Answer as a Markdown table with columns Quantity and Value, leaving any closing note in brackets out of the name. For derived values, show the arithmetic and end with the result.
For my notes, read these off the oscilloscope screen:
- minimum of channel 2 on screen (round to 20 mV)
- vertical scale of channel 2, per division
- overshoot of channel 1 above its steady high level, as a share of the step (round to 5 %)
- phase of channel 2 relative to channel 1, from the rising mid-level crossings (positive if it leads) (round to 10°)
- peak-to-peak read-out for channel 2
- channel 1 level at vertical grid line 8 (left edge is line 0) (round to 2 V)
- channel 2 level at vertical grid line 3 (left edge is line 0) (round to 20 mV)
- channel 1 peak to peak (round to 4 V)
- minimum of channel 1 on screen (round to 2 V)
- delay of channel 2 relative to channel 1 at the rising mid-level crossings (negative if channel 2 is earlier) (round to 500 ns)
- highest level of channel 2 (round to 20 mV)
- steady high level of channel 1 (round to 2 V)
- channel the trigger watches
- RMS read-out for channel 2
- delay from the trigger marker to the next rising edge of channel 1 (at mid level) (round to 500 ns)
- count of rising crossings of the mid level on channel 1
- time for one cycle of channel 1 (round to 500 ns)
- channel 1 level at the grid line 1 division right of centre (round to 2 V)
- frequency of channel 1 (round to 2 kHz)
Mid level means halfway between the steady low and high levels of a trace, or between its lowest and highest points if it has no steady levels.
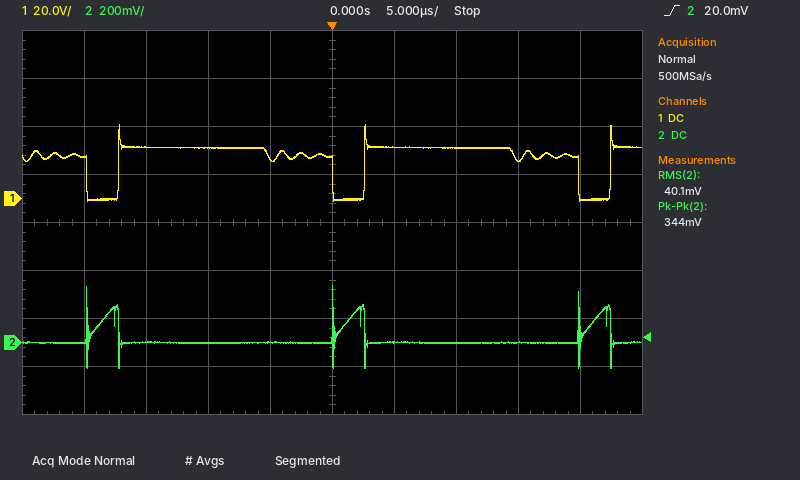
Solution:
| Quantity | Value |
|---|---|
| minimum of channel 2 on screen | -100 mV |
| vertical scale of channel 2, per division | 200 mV |
| overshoot of channel 1 above its steady high level, as a share of the step | 45 % |
| phase of channel 2 relative to channel 1, from the rising mid-level crossings (positive if it leads) | −360° × (-1.5 µs) / 20.0 µs ≈ +27.0°, so +30° to the nearest 10° |
| peak-to-peak read-out for channel 2 | 344 mV |
| channel 1 level at vertical grid line 8 (left edge is line 0) | 16 V |
| channel 2 level at vertical grid line 3 (left edge is line 0) | 0 mV |
| channel 1 peak to peak | 32 V |
| minimum of channel 1 on screen | -2 V |
| delay of channel 2 relative to channel 1 at the rising mid-level crossings (negative if channel 2 is earlier) | -1.5 µs |
| highest level of channel 2 | 240 mV |
| steady high level of channel 1 | 22 V |
| channel the trigger watches | channel 2 |
| RMS read-out for channel 2 | 40.1 mV |
| delay from the trigger marker to the next rising edge of channel 1 (at mid level) | 2.5 µs |
| count of rising crossings of the mid level on channel 1 | 3 |
| time for one cycle of channel 1 | 20.0 µs |
| channel 1 level at the grid line 1 division right of centre | 22 V |
| frequency of channel 1 | 1 / 20.0 µs ≈ 50 kHz |
